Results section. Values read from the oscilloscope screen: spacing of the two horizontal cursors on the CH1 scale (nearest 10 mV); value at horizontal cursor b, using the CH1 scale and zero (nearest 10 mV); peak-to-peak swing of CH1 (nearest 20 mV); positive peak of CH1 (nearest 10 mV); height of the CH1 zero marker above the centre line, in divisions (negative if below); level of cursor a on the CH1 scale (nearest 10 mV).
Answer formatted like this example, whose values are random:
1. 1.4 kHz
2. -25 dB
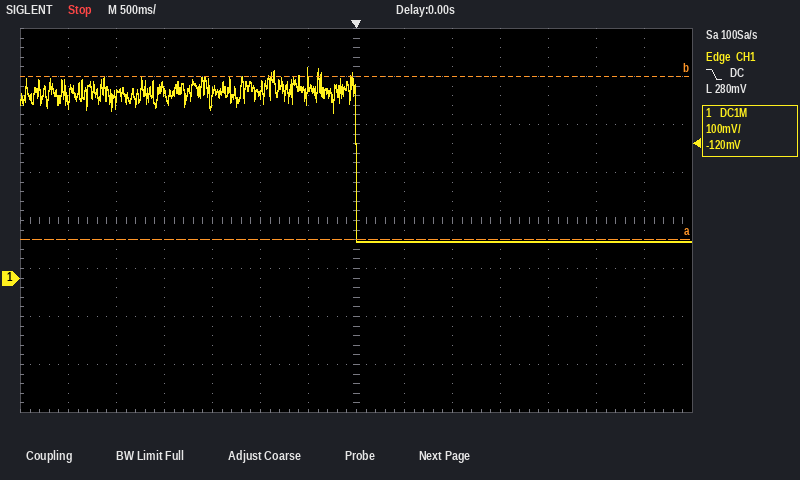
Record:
1. 340 mV
2. 420 mV
3. 360 mV
4. 440 mV
5. -1.2 div
6. 80 mV
